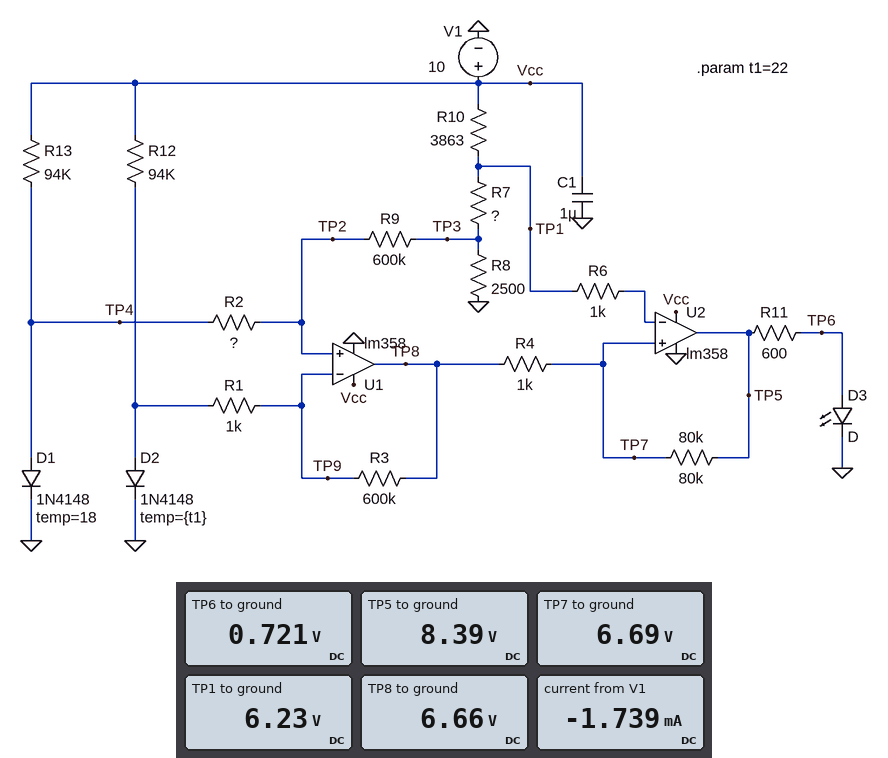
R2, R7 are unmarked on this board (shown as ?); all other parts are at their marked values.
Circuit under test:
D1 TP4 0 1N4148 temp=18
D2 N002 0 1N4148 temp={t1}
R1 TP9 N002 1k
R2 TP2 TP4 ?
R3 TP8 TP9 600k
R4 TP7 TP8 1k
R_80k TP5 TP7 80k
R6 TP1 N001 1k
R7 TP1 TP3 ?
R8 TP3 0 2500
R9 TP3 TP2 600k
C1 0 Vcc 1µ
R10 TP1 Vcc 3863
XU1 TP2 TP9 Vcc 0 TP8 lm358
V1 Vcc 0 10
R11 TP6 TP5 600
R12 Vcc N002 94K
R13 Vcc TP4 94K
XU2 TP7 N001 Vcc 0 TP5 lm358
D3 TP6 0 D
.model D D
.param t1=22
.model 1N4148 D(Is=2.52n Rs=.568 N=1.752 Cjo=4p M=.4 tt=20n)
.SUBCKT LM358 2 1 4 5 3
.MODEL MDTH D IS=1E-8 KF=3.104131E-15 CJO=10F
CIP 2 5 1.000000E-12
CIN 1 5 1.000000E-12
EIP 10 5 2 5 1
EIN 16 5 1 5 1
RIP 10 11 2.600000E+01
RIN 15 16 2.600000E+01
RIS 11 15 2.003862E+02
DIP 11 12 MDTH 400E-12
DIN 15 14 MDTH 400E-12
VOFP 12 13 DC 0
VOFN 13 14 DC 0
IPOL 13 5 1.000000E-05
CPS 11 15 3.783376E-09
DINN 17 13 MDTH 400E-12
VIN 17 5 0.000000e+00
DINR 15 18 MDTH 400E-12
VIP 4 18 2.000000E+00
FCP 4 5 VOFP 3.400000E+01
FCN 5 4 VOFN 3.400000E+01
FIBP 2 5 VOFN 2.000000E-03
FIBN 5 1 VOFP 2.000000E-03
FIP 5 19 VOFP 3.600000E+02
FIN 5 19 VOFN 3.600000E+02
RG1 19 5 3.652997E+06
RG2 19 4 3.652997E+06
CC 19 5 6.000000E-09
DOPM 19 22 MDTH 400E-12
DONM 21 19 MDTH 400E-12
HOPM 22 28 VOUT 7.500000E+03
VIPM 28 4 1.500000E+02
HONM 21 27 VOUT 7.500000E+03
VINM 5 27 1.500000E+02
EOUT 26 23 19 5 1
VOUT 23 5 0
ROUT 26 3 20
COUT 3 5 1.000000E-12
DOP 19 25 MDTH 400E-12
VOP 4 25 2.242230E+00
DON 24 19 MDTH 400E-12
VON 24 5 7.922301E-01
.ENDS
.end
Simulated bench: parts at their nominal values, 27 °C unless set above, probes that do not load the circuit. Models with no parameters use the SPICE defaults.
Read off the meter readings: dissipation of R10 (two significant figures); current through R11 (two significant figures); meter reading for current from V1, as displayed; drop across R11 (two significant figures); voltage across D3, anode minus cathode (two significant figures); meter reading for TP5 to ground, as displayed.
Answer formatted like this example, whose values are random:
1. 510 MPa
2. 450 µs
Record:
1. 3.7 mW
2. 13 mA
3. -1.739 mA
4. 7.7 V
5. 720 mV
6. 8.39 V
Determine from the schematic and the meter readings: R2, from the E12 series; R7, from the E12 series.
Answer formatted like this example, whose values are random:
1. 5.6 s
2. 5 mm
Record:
1. 1.2 kΩ
2. 3.9 kΩ
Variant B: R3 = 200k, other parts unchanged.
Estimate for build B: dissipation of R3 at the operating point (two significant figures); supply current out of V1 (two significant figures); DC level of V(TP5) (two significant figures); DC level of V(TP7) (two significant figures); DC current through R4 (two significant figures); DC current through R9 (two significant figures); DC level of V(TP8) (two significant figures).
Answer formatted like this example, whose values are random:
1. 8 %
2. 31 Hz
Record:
1. 21 µW
2. 1.9 mA
3. -98 mV
4. 2.5 V
5. 33 µA
6. 3.2 µA
7. 2.6 V
